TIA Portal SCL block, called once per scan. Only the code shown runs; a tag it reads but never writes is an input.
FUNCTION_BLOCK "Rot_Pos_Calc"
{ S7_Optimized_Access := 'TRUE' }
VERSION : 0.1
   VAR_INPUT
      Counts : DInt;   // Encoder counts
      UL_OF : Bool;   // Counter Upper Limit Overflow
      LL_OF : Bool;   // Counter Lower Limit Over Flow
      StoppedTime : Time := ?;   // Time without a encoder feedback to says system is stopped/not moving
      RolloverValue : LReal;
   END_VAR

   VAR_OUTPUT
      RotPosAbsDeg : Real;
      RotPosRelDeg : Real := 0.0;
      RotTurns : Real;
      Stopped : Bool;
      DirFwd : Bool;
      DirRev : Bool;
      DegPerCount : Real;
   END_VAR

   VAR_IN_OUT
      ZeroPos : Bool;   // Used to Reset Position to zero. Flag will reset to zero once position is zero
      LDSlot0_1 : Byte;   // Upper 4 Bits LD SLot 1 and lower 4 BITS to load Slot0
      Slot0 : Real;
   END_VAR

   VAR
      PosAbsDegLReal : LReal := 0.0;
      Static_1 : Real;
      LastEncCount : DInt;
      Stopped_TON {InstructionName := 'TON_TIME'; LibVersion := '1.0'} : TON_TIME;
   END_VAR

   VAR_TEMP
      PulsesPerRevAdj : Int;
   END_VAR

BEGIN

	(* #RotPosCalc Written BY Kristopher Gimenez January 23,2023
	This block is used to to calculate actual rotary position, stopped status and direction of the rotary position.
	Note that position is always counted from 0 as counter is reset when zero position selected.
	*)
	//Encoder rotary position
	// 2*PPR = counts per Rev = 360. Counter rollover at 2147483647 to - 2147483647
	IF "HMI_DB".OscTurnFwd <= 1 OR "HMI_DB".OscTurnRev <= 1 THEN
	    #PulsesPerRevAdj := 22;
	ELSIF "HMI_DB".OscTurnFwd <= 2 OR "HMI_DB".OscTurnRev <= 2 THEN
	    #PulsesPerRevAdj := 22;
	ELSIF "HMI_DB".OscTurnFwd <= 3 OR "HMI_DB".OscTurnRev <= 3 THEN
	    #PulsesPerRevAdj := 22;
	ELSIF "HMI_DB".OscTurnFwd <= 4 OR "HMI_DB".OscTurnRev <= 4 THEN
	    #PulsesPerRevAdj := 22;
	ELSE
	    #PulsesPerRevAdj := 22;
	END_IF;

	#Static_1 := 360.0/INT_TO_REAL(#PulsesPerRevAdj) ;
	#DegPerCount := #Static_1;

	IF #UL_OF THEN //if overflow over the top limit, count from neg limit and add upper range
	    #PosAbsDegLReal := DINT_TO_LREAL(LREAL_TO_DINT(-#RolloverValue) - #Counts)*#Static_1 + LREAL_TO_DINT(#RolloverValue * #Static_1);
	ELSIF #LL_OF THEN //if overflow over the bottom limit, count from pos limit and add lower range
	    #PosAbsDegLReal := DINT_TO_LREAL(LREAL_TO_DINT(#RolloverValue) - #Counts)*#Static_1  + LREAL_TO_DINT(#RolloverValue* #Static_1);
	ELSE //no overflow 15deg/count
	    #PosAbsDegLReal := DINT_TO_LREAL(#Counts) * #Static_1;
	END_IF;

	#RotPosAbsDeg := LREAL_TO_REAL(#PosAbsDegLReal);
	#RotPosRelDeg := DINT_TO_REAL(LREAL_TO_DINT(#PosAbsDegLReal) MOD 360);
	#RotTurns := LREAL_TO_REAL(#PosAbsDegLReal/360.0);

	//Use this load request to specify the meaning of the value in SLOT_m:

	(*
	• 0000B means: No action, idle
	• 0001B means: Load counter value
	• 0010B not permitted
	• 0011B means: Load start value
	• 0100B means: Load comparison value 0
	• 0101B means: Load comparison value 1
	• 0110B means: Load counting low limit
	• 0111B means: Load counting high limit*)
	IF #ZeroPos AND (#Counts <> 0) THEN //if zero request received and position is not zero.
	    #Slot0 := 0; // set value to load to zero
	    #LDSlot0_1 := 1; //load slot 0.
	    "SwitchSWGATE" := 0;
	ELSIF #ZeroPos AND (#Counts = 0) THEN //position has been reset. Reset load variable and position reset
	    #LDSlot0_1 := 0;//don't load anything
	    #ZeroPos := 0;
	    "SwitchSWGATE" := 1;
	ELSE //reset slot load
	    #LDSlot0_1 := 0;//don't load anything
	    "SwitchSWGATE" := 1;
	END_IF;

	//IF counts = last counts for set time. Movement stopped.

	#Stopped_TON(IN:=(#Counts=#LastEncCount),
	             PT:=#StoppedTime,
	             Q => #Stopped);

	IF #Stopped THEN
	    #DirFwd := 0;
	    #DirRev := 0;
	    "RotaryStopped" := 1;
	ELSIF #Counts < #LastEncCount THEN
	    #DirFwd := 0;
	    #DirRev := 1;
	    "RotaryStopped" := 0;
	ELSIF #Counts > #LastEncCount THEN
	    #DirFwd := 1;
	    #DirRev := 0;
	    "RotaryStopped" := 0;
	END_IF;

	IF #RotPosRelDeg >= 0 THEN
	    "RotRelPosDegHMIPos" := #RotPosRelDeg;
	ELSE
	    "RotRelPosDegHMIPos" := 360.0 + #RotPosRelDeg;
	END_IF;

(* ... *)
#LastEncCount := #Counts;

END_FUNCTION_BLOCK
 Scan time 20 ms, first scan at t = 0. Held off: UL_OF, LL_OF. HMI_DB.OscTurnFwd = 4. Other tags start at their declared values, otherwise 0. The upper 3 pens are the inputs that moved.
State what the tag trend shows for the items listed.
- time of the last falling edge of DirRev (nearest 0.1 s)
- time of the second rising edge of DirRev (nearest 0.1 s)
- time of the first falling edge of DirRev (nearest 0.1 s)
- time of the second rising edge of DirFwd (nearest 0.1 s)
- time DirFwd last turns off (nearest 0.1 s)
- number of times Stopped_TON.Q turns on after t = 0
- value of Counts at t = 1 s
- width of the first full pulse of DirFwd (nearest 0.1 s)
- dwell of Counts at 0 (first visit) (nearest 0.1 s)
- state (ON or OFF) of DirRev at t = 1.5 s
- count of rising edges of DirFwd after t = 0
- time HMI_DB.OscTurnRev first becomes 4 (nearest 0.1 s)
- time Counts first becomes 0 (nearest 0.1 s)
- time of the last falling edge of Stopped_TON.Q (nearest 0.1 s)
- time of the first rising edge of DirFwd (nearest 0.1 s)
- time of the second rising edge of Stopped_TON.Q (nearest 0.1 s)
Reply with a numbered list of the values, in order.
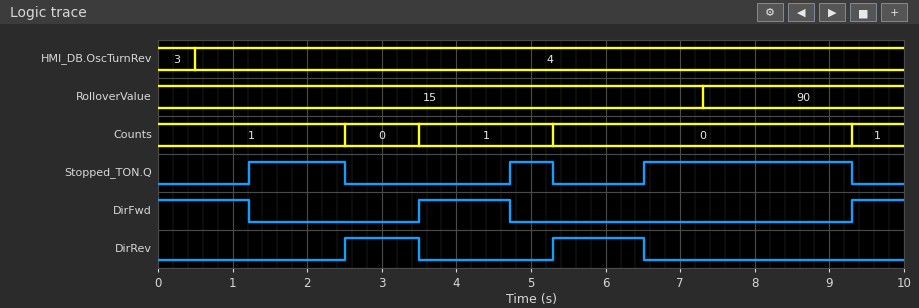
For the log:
1. 6.5 s
2. 5.3 s
3. 3.5 s
4. 9.3 s
5. 4.7 s
6. 3
7. 1
8. 1.2 s
9. 1.0 s
10. OFF
11. 2
12. 0.5 s
13. 2.5 s
14. 9.3 s
15. 3.5 s
16. 4.7 s
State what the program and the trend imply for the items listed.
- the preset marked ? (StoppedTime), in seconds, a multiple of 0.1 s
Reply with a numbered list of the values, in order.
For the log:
1. 1.2 s
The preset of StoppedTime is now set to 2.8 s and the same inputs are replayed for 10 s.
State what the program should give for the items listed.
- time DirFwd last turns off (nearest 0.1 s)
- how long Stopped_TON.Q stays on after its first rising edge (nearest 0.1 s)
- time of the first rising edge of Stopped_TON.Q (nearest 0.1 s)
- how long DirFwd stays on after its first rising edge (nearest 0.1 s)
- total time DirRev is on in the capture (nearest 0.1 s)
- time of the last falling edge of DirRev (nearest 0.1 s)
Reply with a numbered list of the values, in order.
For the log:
1. 5.3 s
2. 1.2 s
3. 8.1 s
4. 1.8 s
5. 3.8 s
6. 8.1 s
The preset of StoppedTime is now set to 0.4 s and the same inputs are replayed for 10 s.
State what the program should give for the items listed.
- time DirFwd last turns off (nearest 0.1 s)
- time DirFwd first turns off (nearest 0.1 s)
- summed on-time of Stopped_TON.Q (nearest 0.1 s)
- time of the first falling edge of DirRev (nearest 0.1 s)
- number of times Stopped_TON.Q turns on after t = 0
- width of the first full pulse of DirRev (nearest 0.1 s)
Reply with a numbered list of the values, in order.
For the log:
1. 9.7 s
2. 0.4 s
3. 7.9 s
4. 2.9 s
5. 5
6. 0.4 s
